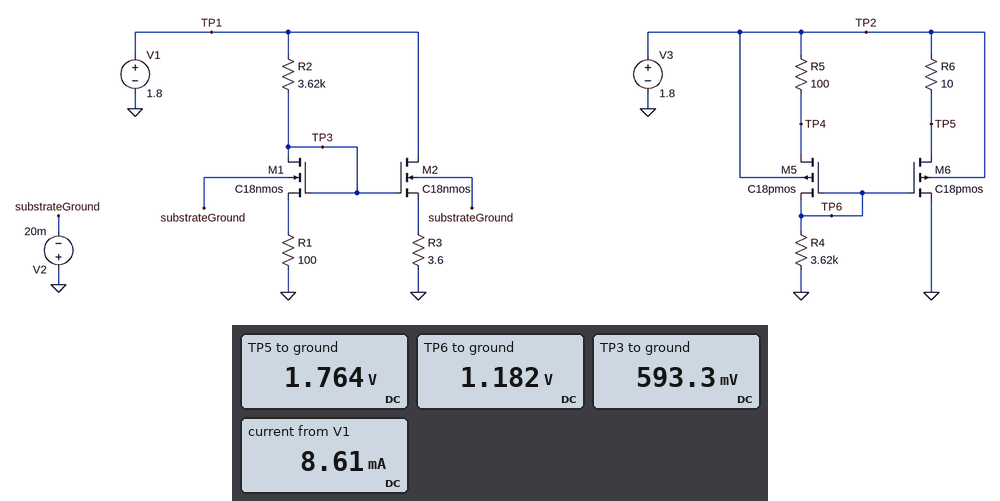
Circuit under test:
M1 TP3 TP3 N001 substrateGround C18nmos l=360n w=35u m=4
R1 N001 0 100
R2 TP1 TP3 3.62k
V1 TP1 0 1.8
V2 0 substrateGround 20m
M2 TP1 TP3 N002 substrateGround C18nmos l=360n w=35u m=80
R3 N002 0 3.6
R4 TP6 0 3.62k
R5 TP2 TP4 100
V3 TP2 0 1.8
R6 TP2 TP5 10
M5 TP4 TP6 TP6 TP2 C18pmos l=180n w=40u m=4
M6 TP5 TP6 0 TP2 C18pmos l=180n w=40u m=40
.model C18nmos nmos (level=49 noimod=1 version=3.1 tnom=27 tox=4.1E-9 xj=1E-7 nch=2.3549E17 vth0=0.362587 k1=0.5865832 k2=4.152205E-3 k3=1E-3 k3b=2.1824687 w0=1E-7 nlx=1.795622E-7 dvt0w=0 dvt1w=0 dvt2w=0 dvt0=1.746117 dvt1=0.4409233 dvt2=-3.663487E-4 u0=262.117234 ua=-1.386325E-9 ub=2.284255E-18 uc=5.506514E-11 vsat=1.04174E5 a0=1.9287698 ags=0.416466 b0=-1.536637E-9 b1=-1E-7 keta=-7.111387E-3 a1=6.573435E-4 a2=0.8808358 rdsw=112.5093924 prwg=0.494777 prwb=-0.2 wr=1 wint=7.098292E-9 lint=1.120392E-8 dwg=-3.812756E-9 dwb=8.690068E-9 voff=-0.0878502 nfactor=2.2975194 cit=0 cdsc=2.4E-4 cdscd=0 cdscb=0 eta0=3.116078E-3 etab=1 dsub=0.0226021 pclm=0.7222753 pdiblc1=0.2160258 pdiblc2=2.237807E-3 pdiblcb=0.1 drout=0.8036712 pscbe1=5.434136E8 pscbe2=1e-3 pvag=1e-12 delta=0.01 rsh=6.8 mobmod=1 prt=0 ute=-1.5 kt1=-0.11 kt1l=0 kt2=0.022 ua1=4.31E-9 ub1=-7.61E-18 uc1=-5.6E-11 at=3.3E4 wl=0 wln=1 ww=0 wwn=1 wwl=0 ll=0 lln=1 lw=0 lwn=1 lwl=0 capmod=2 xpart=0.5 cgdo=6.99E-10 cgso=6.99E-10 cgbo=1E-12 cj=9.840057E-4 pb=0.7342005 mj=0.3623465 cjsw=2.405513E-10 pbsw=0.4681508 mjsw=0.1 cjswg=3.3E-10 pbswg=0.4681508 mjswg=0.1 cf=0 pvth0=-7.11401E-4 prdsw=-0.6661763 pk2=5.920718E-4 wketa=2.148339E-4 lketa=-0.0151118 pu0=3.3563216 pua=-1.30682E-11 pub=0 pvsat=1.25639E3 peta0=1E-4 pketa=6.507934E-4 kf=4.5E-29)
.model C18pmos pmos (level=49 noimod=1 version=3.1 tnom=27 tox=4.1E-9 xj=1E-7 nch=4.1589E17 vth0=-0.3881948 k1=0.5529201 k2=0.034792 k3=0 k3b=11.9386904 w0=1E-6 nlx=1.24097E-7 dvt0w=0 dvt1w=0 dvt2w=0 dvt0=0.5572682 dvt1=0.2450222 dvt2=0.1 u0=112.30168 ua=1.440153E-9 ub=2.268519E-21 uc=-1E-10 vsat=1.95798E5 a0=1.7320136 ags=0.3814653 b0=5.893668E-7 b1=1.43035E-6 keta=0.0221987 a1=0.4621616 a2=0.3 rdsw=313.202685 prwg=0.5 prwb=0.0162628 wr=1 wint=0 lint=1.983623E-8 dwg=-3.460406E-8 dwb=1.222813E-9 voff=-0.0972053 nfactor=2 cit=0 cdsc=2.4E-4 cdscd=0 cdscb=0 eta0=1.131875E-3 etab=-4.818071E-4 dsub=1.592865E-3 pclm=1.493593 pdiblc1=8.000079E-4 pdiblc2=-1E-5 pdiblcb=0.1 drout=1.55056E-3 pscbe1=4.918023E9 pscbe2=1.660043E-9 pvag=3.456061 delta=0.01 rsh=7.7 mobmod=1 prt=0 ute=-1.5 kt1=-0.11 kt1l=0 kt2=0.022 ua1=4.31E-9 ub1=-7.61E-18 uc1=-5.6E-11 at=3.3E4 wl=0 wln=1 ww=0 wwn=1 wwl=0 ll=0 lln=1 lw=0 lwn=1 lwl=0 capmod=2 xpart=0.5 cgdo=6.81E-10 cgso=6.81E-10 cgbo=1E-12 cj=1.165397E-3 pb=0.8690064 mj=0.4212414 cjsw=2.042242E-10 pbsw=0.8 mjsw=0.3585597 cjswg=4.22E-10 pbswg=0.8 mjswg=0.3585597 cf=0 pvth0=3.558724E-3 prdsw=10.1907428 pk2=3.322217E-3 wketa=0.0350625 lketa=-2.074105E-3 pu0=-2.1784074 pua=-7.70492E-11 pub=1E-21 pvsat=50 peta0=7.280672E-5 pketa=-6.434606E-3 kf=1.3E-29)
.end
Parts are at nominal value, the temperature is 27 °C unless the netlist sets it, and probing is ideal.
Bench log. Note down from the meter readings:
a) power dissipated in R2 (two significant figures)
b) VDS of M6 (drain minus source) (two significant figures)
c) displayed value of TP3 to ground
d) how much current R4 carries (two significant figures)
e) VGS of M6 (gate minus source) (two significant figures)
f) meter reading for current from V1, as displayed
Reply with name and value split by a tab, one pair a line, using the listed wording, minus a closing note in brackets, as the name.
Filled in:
power dissipated in R2	400 µW
VDS of M6 (drain minus source)	1.8 V
displayed value of TP3 to ground	593.3 mV
how much current R4 carries	330 µA
VGS of M6 (gate minus source)	1.2 V
meter reading for current from V1, as displayed	8.61 mA
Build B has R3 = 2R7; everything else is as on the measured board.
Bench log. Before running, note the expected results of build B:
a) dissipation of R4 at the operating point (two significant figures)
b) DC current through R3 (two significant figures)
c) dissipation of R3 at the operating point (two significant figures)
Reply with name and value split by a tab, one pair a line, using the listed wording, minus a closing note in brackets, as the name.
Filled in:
dissipation of R4 at the operating point	390 µW
DC current through R3	9.2 mA
dissipation of R3 at the operating point	230 µW
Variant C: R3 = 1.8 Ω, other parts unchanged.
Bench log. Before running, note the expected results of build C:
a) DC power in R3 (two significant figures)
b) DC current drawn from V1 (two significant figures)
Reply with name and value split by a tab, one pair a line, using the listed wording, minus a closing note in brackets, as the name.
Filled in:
DC power in R3	200 µW
DC current drawn from V1	11 mA
